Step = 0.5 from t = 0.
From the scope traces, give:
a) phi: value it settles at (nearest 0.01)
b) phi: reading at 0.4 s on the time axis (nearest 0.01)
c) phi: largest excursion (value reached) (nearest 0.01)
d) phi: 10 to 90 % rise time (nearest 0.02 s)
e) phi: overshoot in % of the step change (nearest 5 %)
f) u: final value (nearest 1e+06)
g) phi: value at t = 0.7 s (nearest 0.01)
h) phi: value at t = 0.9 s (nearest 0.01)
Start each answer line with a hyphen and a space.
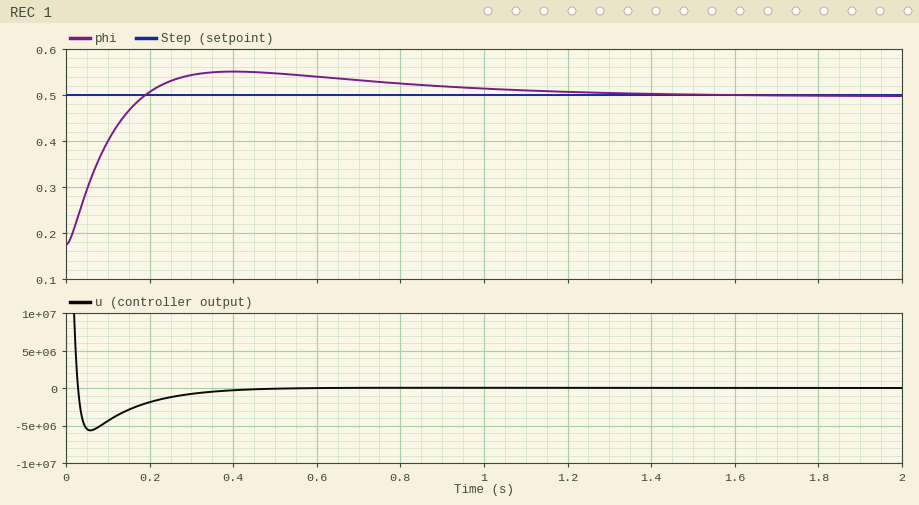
- 0.50
- 0.55
- 0.55
- 0.14 s
- 15 %
- 0
- 0.53
- 0.52
